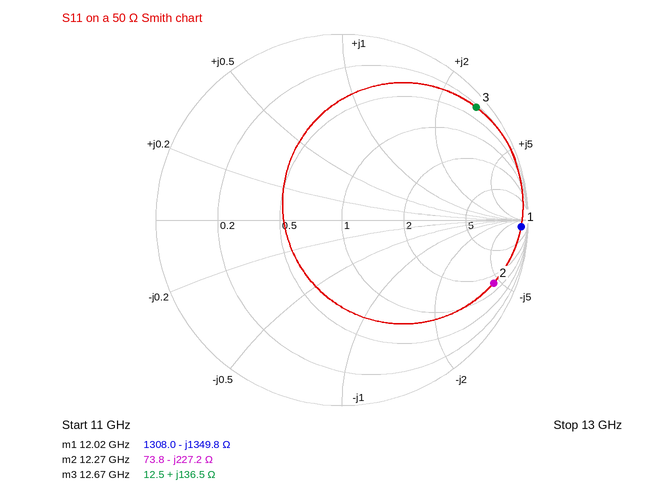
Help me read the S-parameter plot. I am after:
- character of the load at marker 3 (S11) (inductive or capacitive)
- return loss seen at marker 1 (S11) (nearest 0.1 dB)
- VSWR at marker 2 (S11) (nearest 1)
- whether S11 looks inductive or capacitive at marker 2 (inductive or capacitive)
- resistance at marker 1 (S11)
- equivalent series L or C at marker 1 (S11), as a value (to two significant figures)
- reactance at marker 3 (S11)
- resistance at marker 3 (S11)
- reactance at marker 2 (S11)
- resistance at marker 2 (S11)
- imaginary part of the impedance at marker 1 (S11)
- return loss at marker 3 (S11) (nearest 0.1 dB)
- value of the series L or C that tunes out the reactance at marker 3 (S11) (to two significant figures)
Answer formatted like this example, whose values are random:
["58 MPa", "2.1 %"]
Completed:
["inductive", "0.3 dB", "16", "capacitive", "1308.0 Ω", "9.8 fF", "+136.5 Ω", "12.5 Ω", "-227.2 Ω", "73.8 Ω", "-1349.8 Ω", "0.5 dB", "92 fF"]
